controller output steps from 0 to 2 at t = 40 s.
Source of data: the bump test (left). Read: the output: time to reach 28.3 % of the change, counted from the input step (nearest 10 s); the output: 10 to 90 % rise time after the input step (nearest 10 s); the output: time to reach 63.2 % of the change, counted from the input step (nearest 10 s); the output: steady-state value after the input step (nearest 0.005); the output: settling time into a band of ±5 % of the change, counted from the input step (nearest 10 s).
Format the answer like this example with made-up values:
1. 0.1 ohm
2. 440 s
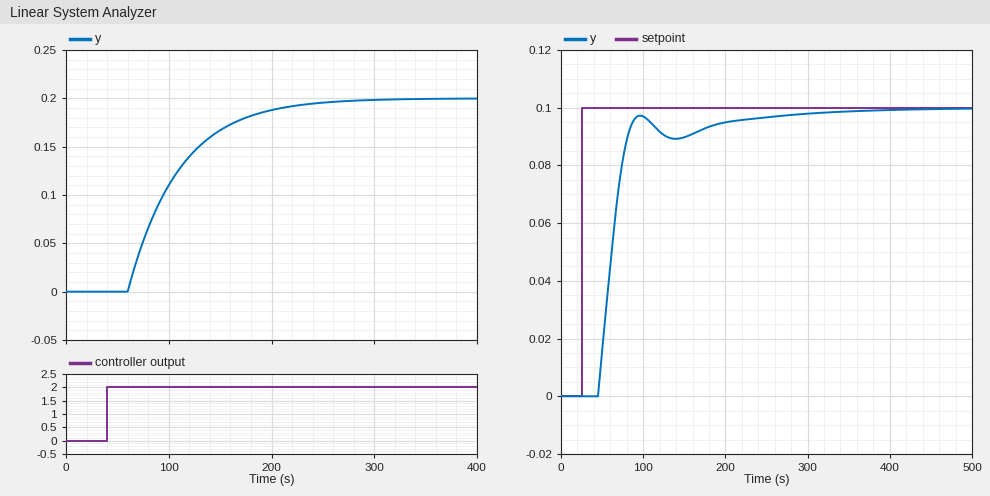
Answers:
1. 40 s
2. 110 s
3. 70 s
4. 0.200
5. 170 s
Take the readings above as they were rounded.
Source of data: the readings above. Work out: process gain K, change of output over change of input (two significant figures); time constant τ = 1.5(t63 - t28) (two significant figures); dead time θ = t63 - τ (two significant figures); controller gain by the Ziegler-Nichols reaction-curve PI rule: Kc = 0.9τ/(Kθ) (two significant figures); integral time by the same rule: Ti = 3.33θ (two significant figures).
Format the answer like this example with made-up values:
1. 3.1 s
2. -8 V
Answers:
1. 0.10
2. 45 s
3. 25 s
4. 16
5. 83 s
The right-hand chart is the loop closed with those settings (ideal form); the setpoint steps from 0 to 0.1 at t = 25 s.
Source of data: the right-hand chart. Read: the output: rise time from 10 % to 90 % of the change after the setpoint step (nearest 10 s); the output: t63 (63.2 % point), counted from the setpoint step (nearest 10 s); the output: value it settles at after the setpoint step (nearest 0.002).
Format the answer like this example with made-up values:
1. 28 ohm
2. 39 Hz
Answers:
1. 30 s
2. 40 s
3. 0.100
